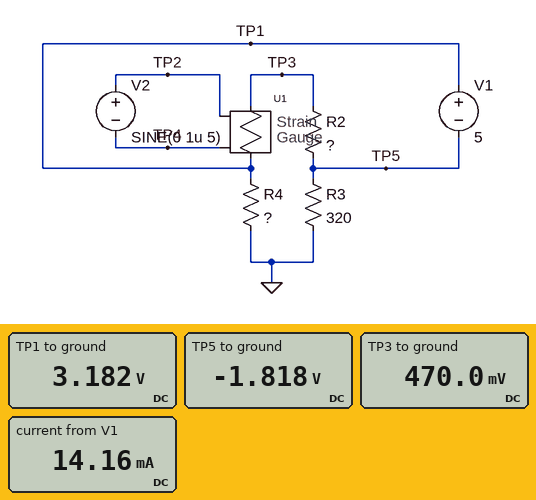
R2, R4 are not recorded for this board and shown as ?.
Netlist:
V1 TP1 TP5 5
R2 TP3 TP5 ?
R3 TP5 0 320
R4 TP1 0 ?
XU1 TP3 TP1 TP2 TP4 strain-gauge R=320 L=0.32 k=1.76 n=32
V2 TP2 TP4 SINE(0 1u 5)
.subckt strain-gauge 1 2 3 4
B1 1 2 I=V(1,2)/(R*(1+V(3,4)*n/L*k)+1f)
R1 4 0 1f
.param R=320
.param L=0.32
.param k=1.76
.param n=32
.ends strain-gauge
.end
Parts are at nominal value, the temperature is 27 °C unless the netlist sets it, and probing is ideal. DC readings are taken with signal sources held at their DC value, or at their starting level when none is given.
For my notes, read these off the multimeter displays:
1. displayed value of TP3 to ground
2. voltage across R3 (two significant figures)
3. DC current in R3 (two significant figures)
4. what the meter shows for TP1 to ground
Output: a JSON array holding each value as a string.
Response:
["470.0 mV", "1.8 V", "5.7 mA", "3.182 V"]
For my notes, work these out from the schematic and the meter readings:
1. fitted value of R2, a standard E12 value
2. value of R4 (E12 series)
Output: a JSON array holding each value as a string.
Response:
["270 Ω", "560 Ω"]
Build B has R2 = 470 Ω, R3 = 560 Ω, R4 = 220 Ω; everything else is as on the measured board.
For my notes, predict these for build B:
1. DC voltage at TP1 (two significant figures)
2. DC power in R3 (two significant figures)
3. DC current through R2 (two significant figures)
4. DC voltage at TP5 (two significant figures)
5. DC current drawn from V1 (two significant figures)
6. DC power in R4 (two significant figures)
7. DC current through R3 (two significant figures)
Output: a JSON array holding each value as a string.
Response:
["1.4 V", "23 mW", "6.3 mA", "-3.6 V", "13 mA", "9.0 mW", "6.4 mA"]
